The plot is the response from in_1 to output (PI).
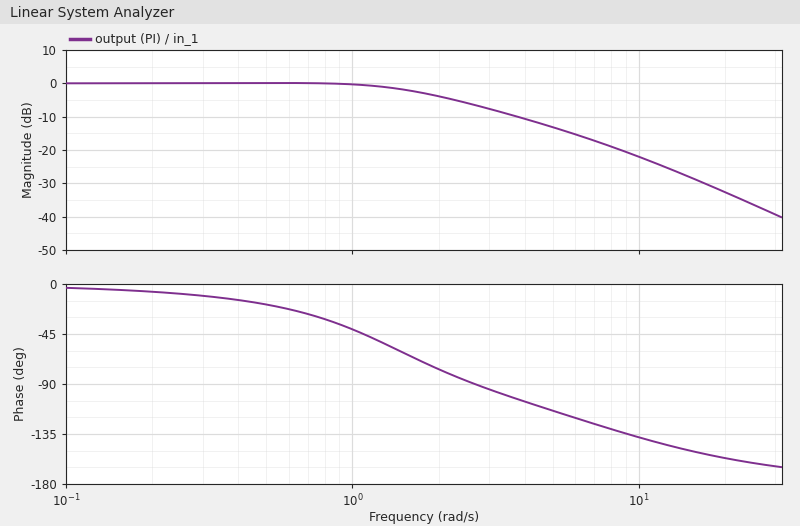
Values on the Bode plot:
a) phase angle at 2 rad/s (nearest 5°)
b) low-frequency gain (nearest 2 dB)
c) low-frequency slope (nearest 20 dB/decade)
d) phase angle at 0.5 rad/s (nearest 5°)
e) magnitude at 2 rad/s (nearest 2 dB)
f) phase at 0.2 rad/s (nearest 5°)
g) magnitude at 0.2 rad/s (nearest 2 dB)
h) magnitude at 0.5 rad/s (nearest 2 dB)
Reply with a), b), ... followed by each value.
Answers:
a) -75°
b) 0 dB
c) 0 dB/decade
d) -20°
e) -4 dB
f) -5°
g) 0 dB
h) 0 dB
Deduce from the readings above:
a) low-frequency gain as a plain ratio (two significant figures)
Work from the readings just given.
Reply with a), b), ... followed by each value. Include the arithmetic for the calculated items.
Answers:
a) 10^(0 / 20) = 1.0
